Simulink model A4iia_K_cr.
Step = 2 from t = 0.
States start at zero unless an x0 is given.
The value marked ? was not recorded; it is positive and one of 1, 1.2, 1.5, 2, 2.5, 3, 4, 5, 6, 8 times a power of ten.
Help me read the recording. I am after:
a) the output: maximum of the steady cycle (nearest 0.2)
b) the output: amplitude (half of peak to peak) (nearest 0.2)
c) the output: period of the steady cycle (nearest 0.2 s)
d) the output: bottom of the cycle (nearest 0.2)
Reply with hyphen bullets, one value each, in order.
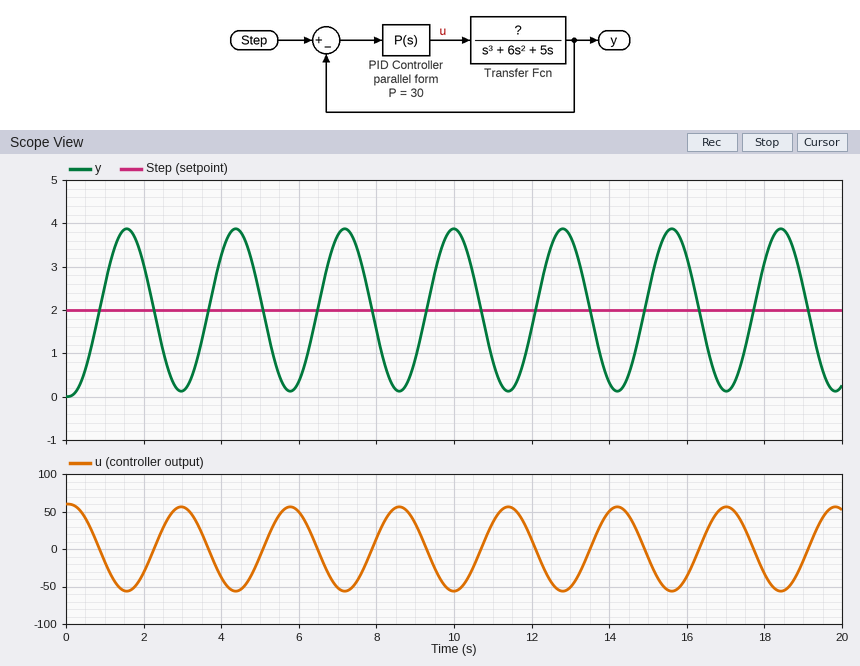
- 3.8
- 1.8
- 2.8 s
- 0.2
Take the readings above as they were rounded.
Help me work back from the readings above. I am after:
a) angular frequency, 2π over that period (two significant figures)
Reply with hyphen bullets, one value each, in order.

- 2.2 rad/s
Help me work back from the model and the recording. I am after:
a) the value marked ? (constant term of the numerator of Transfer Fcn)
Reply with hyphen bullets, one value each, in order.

- 1
